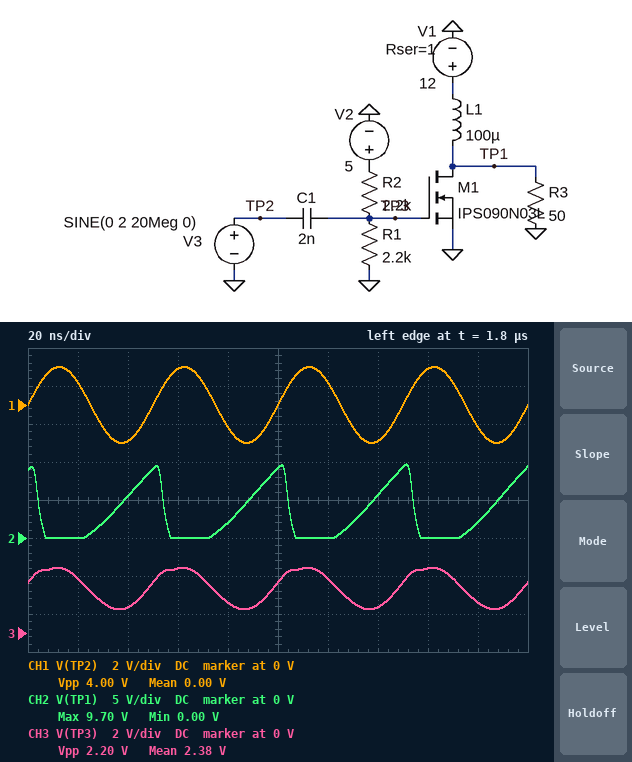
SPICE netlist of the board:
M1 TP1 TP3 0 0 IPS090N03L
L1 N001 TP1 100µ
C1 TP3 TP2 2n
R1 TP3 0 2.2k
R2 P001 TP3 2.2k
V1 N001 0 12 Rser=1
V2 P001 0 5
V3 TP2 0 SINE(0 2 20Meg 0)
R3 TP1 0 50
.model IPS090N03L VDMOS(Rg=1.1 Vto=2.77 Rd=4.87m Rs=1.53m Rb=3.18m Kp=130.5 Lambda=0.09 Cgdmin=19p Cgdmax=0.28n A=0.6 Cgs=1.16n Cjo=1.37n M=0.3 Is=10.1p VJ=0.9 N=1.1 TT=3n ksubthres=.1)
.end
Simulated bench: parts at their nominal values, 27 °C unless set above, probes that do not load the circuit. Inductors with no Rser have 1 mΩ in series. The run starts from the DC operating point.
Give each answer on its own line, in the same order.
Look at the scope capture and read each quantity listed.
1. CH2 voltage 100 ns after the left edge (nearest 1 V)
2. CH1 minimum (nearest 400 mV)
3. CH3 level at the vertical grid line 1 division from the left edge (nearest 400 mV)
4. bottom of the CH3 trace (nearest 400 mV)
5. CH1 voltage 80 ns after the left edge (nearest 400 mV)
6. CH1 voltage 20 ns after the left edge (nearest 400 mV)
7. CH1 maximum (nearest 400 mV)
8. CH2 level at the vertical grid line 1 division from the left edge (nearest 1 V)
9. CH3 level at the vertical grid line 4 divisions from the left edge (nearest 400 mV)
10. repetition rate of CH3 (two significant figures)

9 V
-2.0 V
2.8 V
1.2 V
-1.2 V
1.2 V
2.0 V
0 V
1.6 V
20 MHz
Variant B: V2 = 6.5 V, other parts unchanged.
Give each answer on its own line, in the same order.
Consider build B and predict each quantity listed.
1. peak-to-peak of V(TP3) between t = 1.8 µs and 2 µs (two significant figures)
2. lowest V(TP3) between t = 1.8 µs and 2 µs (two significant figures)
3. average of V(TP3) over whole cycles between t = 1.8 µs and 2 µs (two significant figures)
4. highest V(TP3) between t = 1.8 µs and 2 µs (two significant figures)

1.7 V
2.6 V
3.4 V
4.3 V
